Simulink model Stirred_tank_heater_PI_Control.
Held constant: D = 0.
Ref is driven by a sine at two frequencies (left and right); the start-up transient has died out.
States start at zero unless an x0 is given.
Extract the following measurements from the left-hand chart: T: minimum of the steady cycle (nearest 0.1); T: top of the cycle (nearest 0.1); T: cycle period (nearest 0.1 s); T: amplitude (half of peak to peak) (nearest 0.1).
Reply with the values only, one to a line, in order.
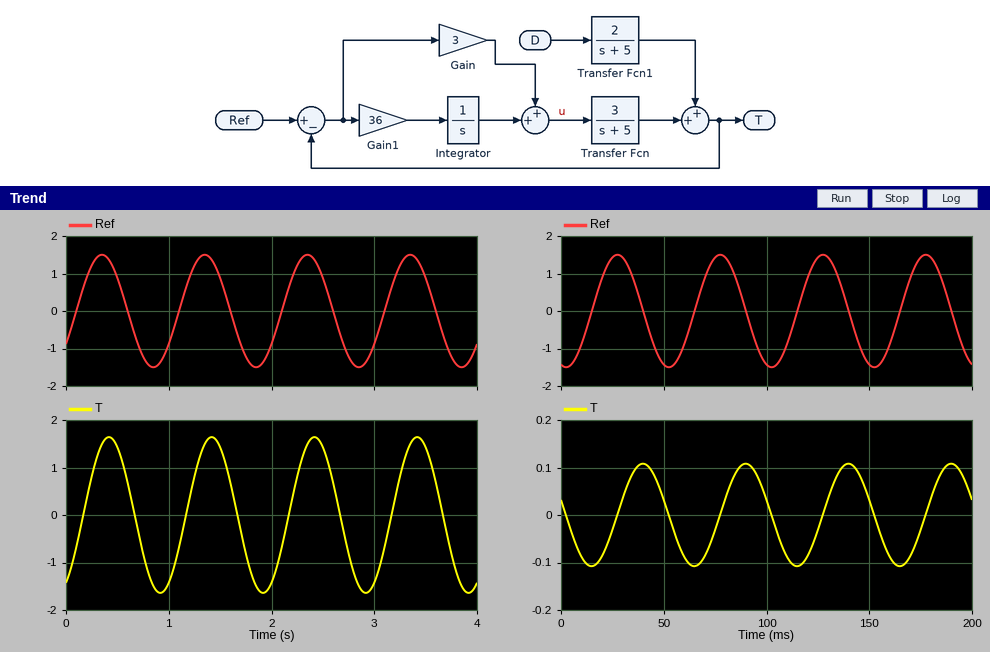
-1.6
1.6
1.0 s
1.6
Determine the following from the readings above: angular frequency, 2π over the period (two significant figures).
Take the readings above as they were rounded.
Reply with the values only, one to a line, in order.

6.3 rad/s
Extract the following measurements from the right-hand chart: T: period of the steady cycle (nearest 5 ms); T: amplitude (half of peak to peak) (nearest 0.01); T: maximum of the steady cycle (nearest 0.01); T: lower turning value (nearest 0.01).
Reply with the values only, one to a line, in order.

50 ms
0.11
0.11
-0.11
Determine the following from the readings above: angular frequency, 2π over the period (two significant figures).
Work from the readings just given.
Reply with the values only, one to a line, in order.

0.13 rad/ms
